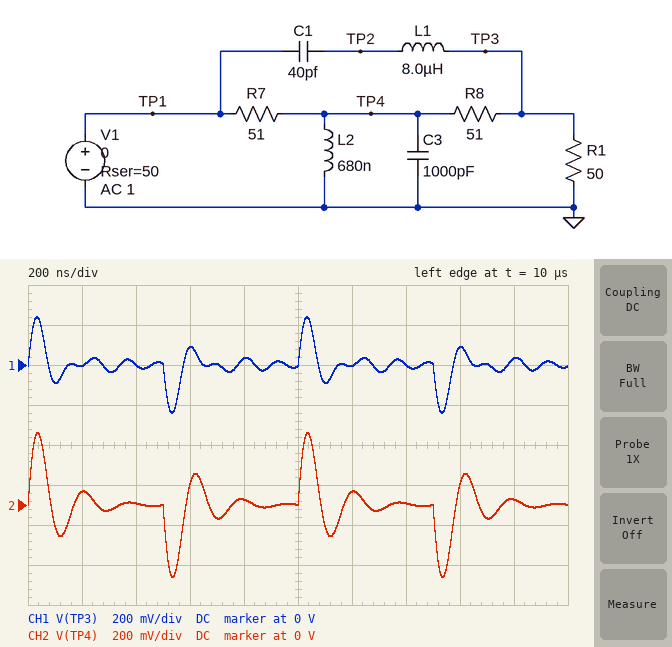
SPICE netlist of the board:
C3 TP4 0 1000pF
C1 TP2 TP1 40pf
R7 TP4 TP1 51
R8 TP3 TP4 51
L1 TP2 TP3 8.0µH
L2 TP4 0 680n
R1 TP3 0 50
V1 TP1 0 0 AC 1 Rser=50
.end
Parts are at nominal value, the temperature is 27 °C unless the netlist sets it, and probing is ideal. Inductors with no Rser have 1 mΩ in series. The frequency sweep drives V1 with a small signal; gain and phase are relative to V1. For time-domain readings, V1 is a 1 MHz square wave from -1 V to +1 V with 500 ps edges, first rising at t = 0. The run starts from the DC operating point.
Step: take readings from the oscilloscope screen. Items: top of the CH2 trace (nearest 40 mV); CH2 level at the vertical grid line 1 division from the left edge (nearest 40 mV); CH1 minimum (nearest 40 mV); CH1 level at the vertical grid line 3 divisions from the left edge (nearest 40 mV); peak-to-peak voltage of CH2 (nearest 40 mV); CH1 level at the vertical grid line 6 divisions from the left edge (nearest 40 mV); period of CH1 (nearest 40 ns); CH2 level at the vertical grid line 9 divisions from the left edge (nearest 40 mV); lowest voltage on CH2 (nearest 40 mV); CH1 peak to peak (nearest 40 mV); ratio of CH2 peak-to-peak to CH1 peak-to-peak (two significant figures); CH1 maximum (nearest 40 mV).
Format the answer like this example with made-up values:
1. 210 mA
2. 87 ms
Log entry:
1. 360 mV
2. 80 mV
3. -240 mV
4. 80 mV
5. 720 mV
6. 0 V
7. 1.00 µs
8. 40 mV
9. -360 mV
10. 480 mV
11. 1.5
12. 240 mV
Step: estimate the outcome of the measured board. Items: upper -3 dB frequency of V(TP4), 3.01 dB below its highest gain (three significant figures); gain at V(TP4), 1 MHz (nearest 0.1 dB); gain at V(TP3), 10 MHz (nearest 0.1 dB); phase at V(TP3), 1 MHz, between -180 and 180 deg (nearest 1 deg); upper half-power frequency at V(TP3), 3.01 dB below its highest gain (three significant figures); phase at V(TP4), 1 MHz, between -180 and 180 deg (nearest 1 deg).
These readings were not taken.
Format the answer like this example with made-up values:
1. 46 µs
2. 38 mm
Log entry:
1. 7.88 MHz
2. -27.3 dB
3. -13.1 dB
4. 86 deg
5. 9.73 MHz
6. 85 deg
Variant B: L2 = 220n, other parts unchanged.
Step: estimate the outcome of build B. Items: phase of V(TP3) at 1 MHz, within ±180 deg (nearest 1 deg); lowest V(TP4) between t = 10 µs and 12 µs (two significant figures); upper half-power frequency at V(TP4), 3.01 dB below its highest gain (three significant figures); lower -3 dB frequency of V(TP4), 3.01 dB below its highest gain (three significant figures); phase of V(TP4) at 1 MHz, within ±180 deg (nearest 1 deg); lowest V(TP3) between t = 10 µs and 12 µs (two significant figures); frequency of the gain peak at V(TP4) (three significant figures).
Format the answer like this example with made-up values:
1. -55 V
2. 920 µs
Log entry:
1. 89 deg
2. -240 mV
3. 12.4 MHz
4. 9.27 MHz
5. 88 deg
6. -180 mV
7. 10.7 MHz
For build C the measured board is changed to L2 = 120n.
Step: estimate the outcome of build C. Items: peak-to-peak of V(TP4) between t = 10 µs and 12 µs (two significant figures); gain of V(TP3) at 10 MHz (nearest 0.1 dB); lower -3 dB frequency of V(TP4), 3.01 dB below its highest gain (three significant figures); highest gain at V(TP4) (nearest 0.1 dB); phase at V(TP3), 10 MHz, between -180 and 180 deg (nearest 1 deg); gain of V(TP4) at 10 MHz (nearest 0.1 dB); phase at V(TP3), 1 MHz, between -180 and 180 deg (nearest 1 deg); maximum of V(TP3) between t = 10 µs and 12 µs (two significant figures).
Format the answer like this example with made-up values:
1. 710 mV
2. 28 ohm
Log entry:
1. 370 mV
2. -22.6 dB
3. 13.0 MHz
4. -6.0 dB
5. -27 deg
6. -17.3 dB
7. 89 deg
8. 140 mV
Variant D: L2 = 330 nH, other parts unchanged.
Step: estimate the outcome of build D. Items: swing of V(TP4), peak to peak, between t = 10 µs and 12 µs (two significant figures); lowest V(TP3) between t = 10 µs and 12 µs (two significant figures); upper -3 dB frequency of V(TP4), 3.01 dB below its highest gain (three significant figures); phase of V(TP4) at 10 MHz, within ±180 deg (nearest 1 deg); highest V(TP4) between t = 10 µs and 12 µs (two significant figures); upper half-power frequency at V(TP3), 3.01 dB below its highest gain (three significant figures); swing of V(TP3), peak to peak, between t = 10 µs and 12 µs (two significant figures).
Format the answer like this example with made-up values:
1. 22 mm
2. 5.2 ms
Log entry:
1. 560 mV
2. -200 mV
3. 10.5 MHz
4. -36 deg
5. 280 mV
6. 9.65 MHz
7. 400 mV
